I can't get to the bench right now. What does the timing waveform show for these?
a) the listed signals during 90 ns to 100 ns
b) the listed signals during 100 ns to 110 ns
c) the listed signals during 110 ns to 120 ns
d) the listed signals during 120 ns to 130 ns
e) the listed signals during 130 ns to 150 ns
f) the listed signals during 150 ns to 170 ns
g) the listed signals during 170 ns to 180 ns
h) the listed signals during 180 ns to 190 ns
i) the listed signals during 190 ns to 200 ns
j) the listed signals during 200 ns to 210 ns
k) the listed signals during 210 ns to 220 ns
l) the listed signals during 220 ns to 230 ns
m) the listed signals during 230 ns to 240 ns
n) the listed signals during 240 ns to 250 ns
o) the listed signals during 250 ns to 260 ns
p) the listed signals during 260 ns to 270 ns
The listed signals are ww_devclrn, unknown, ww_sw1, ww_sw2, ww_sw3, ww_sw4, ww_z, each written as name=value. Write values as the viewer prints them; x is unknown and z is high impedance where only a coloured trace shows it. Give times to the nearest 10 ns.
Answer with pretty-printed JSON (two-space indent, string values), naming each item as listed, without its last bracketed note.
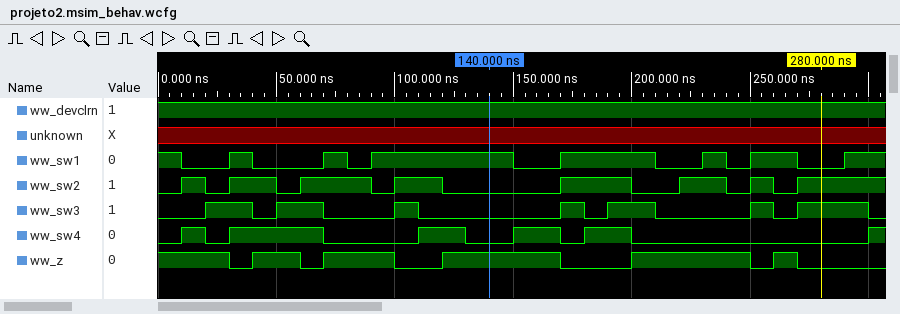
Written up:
{
  "the listed signals during 90 ns to 100 ns": "ww_devclrn=1, unknown=x, ww_sw1=1, ww_sw2=0, ww_sw3=0, ww_sw4=0, ww_z=1",
  "the listed signals during 100 ns to 110 ns": "ww_devclrn=1, unknown=x, ww_sw1=1, ww_sw2=1, ww_sw3=1, ww_sw4=0, ww_z=0",
  "the listed signals during 110 ns to 120 ns": "ww_devclrn=1, unknown=x, ww_sw1=1, ww_sw2=1, ww_sw3=0, ww_sw4=1, ww_z=0",
  "the listed signals during 120 ns to 130 ns": "ww_devclrn=1, unknown=x, ww_sw1=1, ww_sw2=0, ww_sw3=0, ww_sw4=1, ww_z=1",
  "the listed signals during 130 ns to 150 ns": "ww_devclrn=1, unknown=x, ww_sw1=1, ww_sw2=0, ww_sw3=0, ww_sw4=0, ww_z=1",
  "the listed signals during 150 ns to 170 ns": "ww_devclrn=1, unknown=x, ww_sw1=0, ww_sw2=0, ww_sw3=0, ww_sw4=1, ww_z=1",
  "the listed signals during 170 ns to 180 ns": "ww_devclrn=1, unknown=x, ww_sw1=1, ww_sw2=1, ww_sw3=1, ww_sw4=0, ww_z=0",
  "the listed signals during 180 ns to 190 ns": "ww_devclrn=1, unknown=x, ww_sw1=1, ww_sw2=1, ww_sw3=0, ww_sw4=1, ww_z=0",
  "the listed signals during 190 ns to 200 ns": "ww_devclrn=1, unknown=x, ww_sw1=1, ww_sw2=1, ww_sw3=1, ww_sw4=1, ww_z=0",
  "the listed signals during 200 ns to 210 ns": "ww_devclrn=1, unknown=x, ww_sw1=1, ww_sw2=0, ww_sw3=1, ww_sw4=0, ww_z=1",
  "the listed signals during 210 ns to 220 ns": "ww_devclrn=1, unknown=x, ww_sw1=0, ww_sw2=0, ww_sw3=0, ww_sw4=0, ww_z=1",
  "the listed signals during 220 ns to 230 ns": "ww_devclrn=1, unknown=x, ww_sw1=0, ww_sw2=1, ww_sw3=0, ww_sw4=0, ww_z=1",
  "the listed signals during 230 ns to 240 ns": "ww_devclrn=1, unknown=x, ww_sw1=1, ww_sw2=1, ww_sw3=0, ww_sw4=0, ww_z=1",
  "the listed signals during 240 ns to 250 ns": "ww_devclrn=1, unknown=x, ww_sw1=0, ww_sw2=0, ww_sw3=0, ww_sw4=0, ww_z=1",
  "the listed signals during 250 ns to 260 ns": "ww_devclrn=1, unknown=x, ww_sw1=1, ww_sw2=1, ww_sw3=1, ww_sw4=0, ww_z=0",
  "the listed signals during 260 ns to 270 ns": "ww_devclrn=1, unknown=x, ww_sw1=1, ww_sw2=0, ww_sw3=0, ww_sw4=0, ww_z=1"
}
